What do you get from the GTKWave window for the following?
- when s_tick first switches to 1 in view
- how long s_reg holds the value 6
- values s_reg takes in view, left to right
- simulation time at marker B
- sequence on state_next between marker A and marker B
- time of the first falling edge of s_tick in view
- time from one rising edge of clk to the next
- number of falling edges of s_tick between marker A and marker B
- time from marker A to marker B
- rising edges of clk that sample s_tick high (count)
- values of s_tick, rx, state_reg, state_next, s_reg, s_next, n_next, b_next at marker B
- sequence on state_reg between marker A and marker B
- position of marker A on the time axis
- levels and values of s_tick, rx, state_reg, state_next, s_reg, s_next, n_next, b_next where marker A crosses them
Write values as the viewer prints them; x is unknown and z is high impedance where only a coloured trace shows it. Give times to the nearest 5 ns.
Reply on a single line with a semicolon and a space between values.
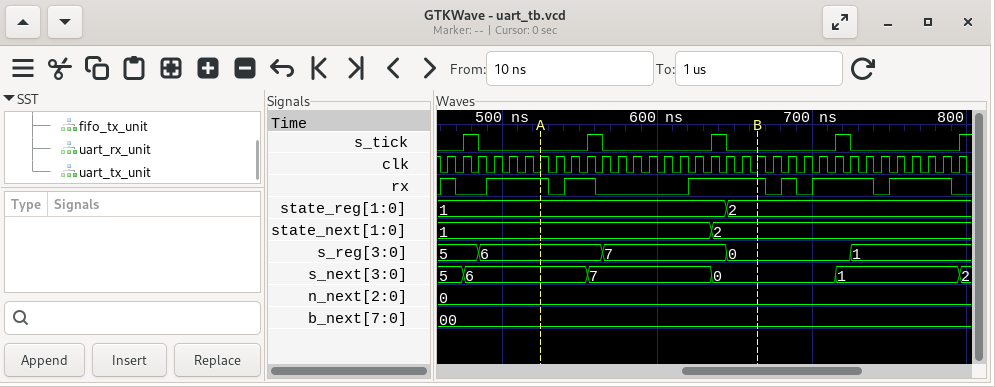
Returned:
475 ns; 80 ns; 5, 6, 7, 0, 1; 665 ns; 1, 2; 485 ns; 10 ns; 2; 140 ns; 4; s_tick=0, rx=1, state_reg=2, state_next=2, s_reg=0, s_next=0, n_next=0, b_next=00; 1, 2; 525 ns; s_tick=0, rx=1, state_reg=1, state_next=1, s_reg=6, s_next=6, n_next=0, b_next=00
